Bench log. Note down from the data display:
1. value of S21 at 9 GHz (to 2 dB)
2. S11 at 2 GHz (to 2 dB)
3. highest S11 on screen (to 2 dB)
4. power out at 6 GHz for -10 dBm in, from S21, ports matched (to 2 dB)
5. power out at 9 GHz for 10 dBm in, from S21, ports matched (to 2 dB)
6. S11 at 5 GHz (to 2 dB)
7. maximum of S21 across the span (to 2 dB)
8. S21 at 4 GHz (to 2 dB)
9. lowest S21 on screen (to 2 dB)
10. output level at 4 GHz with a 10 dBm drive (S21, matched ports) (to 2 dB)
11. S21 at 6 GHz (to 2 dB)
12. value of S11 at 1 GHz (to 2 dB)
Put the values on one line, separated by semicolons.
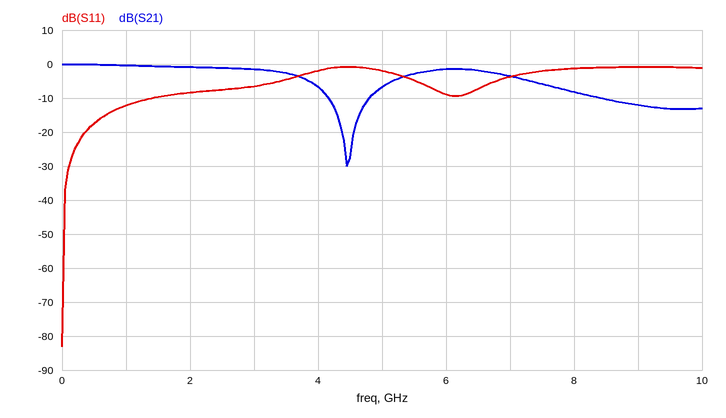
-12 dB; -8 dB; 0 dB; -12 dBm; -2 dBm; -2 dB; 0 dB; -6 dB; -30 dB; 4 dBm; -2 dB; -12 dB
